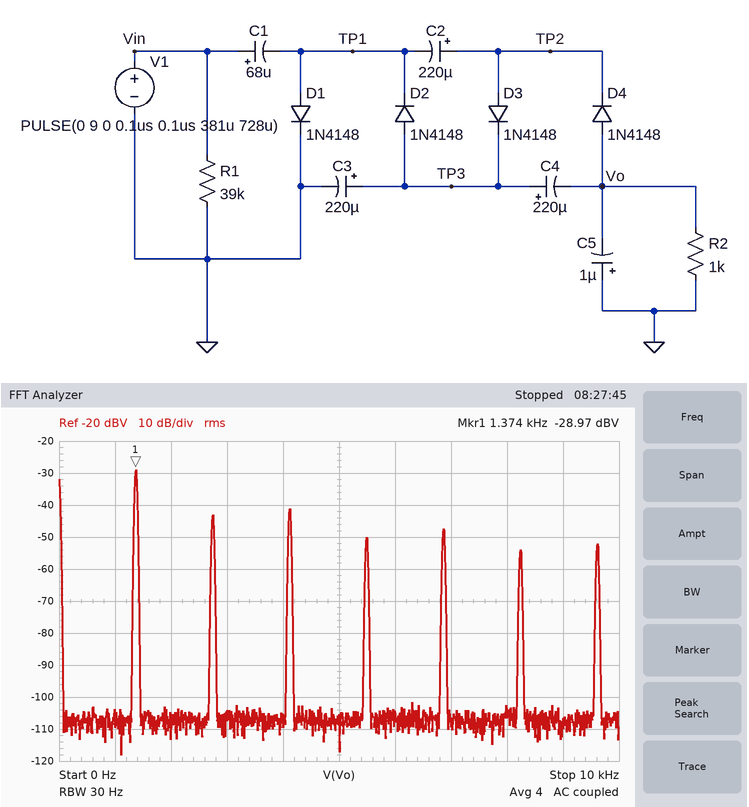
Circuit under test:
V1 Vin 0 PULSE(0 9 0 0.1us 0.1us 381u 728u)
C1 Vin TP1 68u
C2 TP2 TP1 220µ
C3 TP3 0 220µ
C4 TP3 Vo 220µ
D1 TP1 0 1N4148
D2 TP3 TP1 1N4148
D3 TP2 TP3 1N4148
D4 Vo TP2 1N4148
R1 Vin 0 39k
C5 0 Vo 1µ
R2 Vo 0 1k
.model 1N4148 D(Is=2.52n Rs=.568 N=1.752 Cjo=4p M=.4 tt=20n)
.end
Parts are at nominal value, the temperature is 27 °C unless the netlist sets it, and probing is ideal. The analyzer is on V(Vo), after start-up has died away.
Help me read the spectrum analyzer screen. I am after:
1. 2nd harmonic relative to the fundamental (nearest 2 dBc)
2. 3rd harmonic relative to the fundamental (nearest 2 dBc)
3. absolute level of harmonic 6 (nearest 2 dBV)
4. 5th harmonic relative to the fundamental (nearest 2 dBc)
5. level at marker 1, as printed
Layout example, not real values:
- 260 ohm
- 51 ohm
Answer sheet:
- -14 dBc
- -12 dBc
- -54 dBV
- -18 dBc
- -28.97 dBV
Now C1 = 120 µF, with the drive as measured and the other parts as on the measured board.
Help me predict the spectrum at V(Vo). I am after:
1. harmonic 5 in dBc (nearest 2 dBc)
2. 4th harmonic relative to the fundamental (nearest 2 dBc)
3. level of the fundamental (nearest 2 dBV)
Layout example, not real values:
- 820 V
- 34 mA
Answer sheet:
- -20 dBc
- -22 dBc
- -30 dBV
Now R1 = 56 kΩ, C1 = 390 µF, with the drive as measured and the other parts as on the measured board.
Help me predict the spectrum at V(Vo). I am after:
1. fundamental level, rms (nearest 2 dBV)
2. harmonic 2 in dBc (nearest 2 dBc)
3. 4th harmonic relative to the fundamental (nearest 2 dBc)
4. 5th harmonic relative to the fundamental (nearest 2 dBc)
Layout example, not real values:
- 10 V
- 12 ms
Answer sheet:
- -30 dBV
- -18 dBc
- -26 dBc
- -24 dBc
